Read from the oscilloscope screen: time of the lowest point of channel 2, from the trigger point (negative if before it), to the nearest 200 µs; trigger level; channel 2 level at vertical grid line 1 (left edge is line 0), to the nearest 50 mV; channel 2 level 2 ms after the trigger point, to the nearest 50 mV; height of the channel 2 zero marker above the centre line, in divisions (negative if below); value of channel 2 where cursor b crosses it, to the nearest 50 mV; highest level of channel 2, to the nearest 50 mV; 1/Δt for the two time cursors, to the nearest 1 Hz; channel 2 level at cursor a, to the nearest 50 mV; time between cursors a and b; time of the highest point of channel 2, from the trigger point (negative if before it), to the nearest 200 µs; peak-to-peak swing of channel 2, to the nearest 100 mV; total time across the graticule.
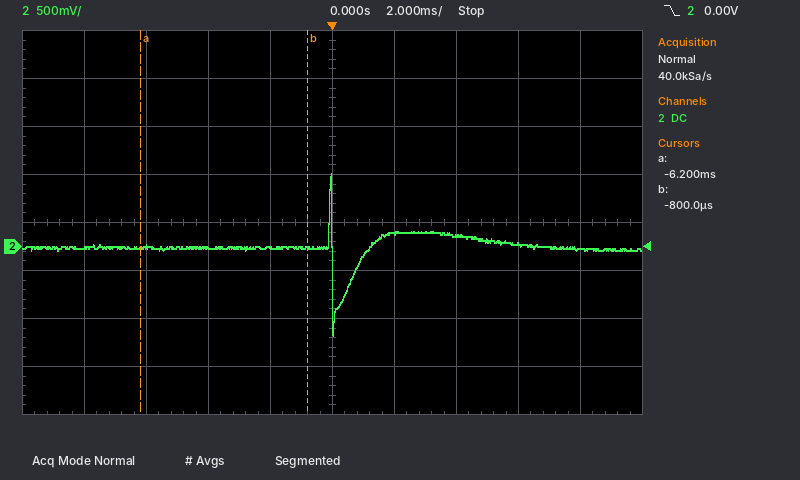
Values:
0.0 ms
0.00 V
0 mV
150 mV
-0.5 div
0 mV
750 mV
185 Hz
0 mV
5.4 ms
0.0 ms
1.70 V
20 ms
